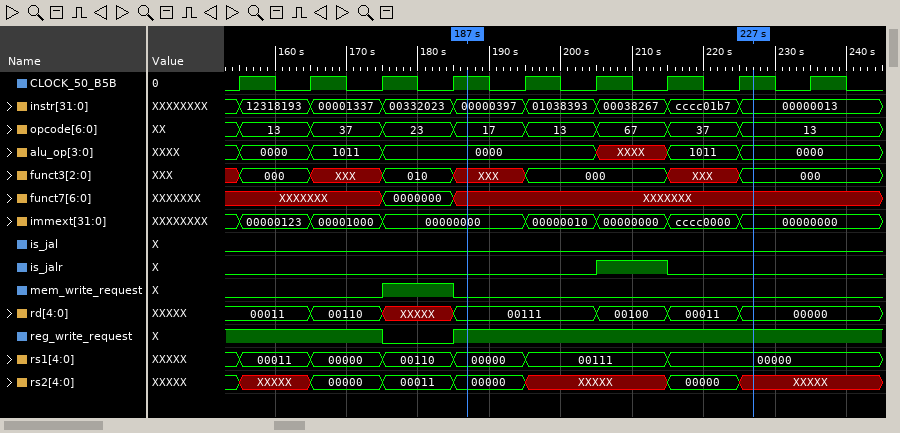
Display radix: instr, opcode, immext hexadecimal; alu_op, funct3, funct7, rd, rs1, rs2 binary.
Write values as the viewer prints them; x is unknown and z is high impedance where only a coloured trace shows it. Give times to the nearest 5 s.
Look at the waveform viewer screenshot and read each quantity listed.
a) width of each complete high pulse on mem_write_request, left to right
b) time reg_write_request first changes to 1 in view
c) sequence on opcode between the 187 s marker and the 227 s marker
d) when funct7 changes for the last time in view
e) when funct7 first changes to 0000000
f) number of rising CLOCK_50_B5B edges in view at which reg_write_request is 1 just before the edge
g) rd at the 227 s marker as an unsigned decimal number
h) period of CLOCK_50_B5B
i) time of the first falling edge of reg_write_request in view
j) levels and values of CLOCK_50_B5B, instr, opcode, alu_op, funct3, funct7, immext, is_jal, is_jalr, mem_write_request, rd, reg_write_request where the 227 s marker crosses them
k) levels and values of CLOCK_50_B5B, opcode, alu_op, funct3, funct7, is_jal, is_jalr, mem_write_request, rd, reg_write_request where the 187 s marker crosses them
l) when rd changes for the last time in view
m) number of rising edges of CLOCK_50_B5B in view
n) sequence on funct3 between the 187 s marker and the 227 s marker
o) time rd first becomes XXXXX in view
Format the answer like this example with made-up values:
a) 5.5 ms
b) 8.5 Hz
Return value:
a) 10 s
b) 185 s
c) 17, 13, 67, 37, 13
d) 185 s
e) 175 s
f) 8
g) 0
h) 10 s
i) 175 s
j) CLOCK_50_B5B=1, instr=00000013, opcode=13, alu_op=0000, funct3=000, funct7=XXXXXXX, immext=00000000, is_jal=0, is_jalr=0, mem_write_request=0, rd=00000, reg_write_request=1
k) CLOCK_50_B5B=1, opcode=17, alu_op=0000, funct3=XXX, funct7=XXXXXXX, is_jal=0, is_jalr=0, mem_write_request=0, rd=00111, reg_write_request=1
l) 225 s
m) 9
n) XXX, 000, XXX, 000
o) 175 s
